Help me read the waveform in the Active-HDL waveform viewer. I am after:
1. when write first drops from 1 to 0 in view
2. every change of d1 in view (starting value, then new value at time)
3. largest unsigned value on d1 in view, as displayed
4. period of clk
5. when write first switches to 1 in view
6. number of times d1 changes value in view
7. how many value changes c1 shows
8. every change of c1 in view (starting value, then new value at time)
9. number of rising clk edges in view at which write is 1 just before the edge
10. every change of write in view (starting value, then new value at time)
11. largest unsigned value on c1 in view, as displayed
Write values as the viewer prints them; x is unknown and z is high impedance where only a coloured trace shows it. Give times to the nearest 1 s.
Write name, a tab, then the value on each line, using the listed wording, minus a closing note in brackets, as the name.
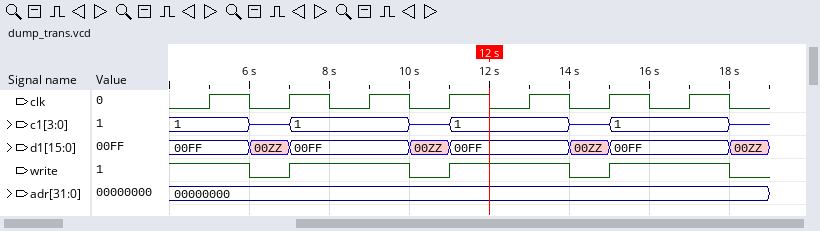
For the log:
when write first drops from 1 to 0 in view	6 s
every change of d1 in view	00FF, 00ZZ at 6 s, 00FF at 7 s, 00ZZ at 10 s, 00FF at 11 s, 00ZZ at 14 s, 00FF at 15 s, 00ZZ at 18 s
largest unsigned value on d1 in view, as displayed	00FF
period of clk	2 s
when write first switches to 1 in view	7 s
number of times d1 changes value in view	7
how many value changes c1 shows	7
every change of c1 in view	1, z at 6 s, 1 at 7 s, z at 10 s, 1 at 11 s, z at 14 s, 1 at 15 s, z at 18 s
number of rising clk edges in view at which write is 1 just before the edge	4
every change of write in view	1, 0 at 6 s, 1 at 7 s, 0 at 10 s, 1 at 11 s, 0 at 14 s, 1 at 15 s, 0 at 18 s
largest unsigned value on c1 in view, as displayed	1
